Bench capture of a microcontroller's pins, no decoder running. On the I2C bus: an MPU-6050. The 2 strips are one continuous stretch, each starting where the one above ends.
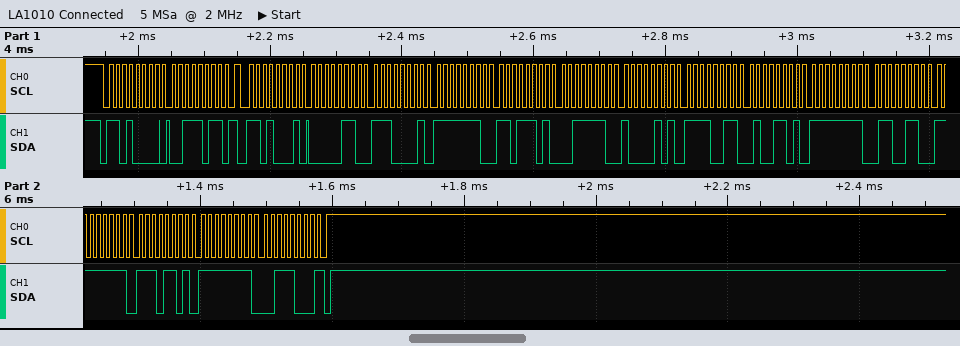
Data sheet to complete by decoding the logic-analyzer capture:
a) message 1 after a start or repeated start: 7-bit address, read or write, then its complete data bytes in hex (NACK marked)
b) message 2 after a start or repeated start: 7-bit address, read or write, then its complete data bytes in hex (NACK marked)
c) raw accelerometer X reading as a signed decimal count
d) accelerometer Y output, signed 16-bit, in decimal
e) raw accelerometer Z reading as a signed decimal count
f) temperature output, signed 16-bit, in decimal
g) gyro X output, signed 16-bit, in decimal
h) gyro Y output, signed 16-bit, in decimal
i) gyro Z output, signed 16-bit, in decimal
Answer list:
0x68 write: 3B
0x68 read: 06 E1 FE DD 3E 85 F3 4D FF 66 FF ED FF 38 NACK
1761
-291
16005
-3251
-154
-19
-200
